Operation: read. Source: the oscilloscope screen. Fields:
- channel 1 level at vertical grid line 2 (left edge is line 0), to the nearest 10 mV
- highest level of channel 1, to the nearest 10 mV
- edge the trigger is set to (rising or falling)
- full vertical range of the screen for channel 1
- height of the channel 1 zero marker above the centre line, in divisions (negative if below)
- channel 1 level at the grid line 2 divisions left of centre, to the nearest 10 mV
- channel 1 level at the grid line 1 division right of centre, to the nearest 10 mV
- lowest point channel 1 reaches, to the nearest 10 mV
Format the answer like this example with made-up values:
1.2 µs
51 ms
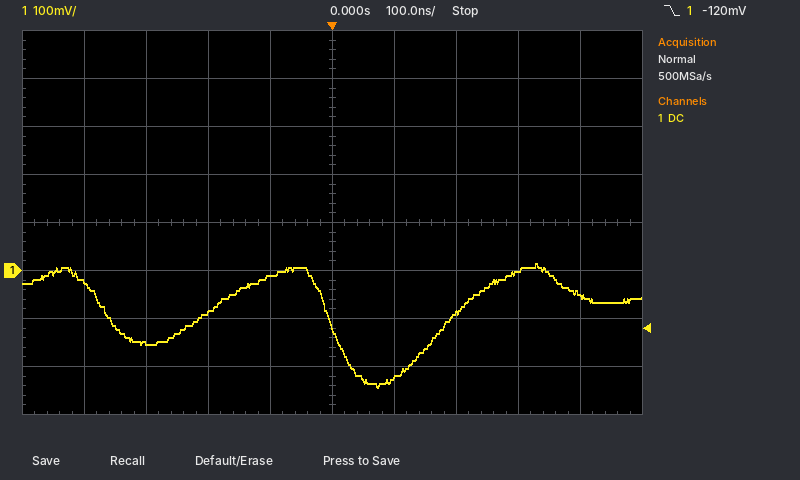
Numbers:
-150 mV
10 mV
falling
800 mV
-1.0 div
-90 mV
-220 mV
-240 mV
